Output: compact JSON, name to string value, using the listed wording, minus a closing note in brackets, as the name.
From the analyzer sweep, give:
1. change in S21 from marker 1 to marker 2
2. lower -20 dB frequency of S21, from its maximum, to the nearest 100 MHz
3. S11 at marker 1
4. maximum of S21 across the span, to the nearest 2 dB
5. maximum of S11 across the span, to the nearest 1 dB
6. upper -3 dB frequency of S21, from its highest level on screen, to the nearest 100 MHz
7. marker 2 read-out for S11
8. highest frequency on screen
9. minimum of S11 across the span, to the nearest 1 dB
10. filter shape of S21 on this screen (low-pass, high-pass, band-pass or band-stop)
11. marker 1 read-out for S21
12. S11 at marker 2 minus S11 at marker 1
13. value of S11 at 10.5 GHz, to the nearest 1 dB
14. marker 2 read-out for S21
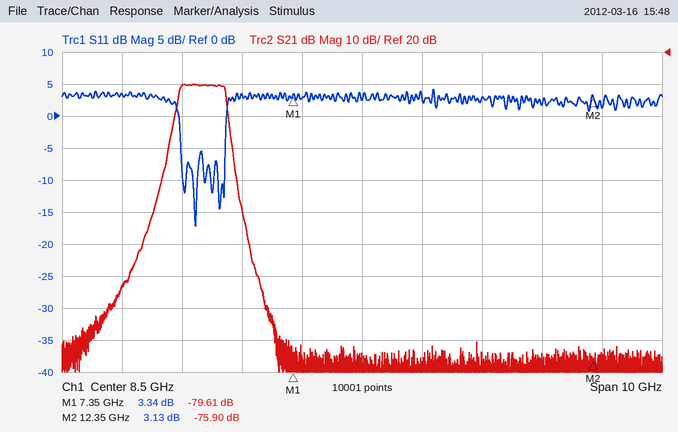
{"change in S21 from marker 1 to marker 2": "3.71 dB", "lower -20 dB frequency of S21, from its maximum, to the nearest 100 MHz": "5.3 GHz", "S11 at marker 1": "3.34 dB", "maximum of S21 across the span, to the nearest 2 dB": "10 dB", "maximum of S11 across the span, to the nearest 1 dB": "4 dB", "upper -3 dB frequency of S21, from its highest level on screen, to the nearest 100 MHz": "6.2 GHz", "marker 2 read-out for S11": "3.13 dB", "highest frequency on screen": "13.5 GHz", "minimum of S11 across the span, to the nearest 1 dB": "-17 dB", "filter shape of S21 on this screen": "band-pass", "marker 1 read-out for S21": "-79.61 dB", "S11 at marker 2 minus S11 at marker 1": "-0.21 dB", "value of S11 at 10.5 GHz, to the nearest 1 dB": "3 dB", "marker 2 read-out for S21": "-75.90 dB"}
